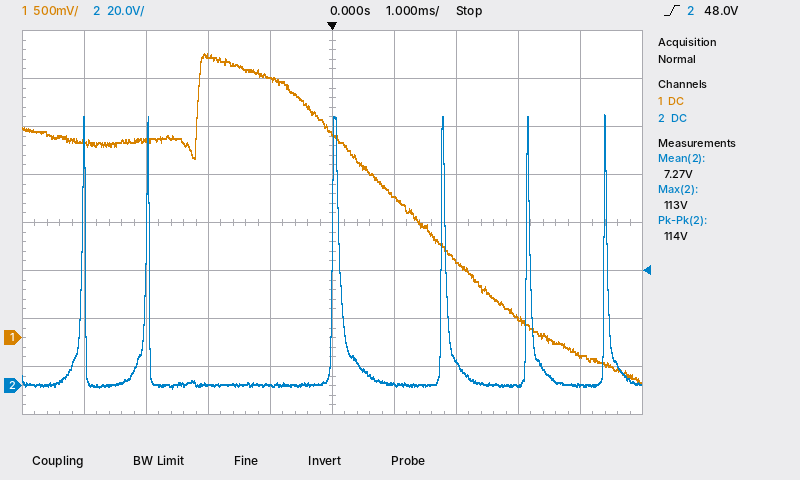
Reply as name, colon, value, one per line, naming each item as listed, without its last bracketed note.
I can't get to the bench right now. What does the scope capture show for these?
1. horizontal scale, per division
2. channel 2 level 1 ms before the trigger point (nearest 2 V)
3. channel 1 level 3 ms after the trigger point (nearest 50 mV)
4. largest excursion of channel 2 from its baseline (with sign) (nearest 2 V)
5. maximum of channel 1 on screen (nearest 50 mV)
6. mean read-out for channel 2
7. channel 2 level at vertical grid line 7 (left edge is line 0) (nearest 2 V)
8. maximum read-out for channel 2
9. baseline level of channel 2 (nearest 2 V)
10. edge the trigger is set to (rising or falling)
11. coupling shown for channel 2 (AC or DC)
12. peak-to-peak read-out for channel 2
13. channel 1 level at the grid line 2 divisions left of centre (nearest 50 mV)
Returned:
horizontal scale, per division: 1 ms
channel 2 level 1 ms before the trigger point: 0 V
channel 1 level 3 ms after the trigger point: 200 mV
largest excursion of channel 2 from its baseline (with sign): +112 V
maximum of channel 1 on screen: 2.95 V
mean read-out for channel 2: 7.27 V
channel 2 level at vertical grid line 7 (left edge is line 0): 10 V
maximum read-out for channel 2: 113 V
baseline level of channel 2: 0 V
edge the trigger is set to: rising
coupling shown for channel 2: DC
peak-to-peak read-out for channel 2: 114 V
channel 1 level at the grid line 2 divisions left of centre: 2.95 V
